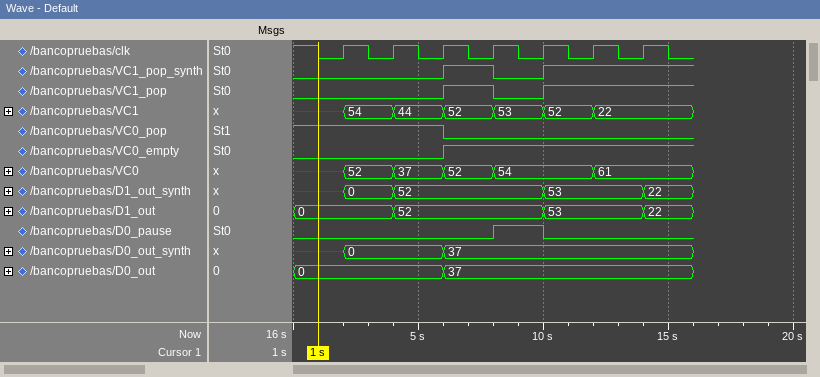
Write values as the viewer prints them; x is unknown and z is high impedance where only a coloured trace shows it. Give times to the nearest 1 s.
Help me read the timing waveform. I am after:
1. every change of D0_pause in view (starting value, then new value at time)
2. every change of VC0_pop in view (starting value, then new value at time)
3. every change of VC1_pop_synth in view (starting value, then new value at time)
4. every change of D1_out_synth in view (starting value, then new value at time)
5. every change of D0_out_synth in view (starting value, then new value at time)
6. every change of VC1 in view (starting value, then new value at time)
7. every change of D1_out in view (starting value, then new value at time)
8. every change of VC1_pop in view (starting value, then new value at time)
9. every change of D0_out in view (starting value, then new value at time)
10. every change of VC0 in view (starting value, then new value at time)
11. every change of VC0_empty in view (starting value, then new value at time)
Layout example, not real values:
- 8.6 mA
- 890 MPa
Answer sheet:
- 0, 1 at 8 s, 0 at 10 s
- 1, 0 at 6 s
- 0, 1 at 6 s, 0 at 8 s, 1 at 10 s
- x, 0 at 2 s, 52 at 4 s, 53 at 10 s, 22 at 14 s
- x, 0 at 2 s, 37 at 6 s
- x, 54 at 2 s, 44 at 4 s, 52 at 6 s, 53 at 8 s, 52 at 10 s, 22 at 12 s
- 0, 52 at 4 s, 53 at 10 s, 22 at 14 s
- 0, 1 at 6 s, 0 at 8 s, 1 at 10 s
- 0, 37 at 6 s
- x, 52 at 2 s, 37 at 4 s, 52 at 6 s, 54 at 8 s, 61 at 12 s
- 0, 1 at 6 s
